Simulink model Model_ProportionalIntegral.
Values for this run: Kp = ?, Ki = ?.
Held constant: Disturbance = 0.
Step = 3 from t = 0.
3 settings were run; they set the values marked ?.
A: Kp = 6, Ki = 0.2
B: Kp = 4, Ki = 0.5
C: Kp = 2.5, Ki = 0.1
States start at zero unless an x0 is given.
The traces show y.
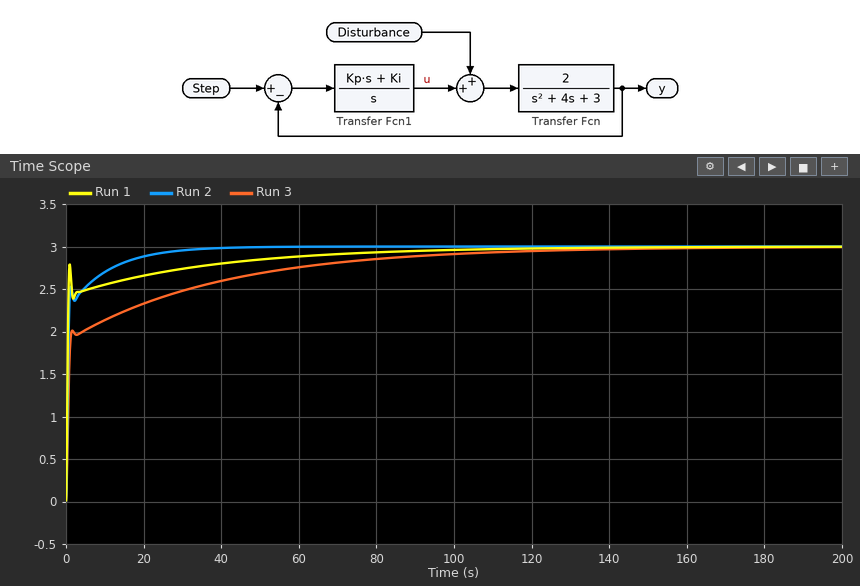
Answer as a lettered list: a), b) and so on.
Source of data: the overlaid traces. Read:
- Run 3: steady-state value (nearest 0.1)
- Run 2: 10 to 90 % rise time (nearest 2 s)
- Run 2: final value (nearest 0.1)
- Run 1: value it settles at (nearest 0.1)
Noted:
a) 3.0
b) 10 s
c) 3.0
d) 3.0
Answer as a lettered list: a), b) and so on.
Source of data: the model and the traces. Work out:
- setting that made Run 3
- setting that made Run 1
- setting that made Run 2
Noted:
a) C
b) A
c) B
